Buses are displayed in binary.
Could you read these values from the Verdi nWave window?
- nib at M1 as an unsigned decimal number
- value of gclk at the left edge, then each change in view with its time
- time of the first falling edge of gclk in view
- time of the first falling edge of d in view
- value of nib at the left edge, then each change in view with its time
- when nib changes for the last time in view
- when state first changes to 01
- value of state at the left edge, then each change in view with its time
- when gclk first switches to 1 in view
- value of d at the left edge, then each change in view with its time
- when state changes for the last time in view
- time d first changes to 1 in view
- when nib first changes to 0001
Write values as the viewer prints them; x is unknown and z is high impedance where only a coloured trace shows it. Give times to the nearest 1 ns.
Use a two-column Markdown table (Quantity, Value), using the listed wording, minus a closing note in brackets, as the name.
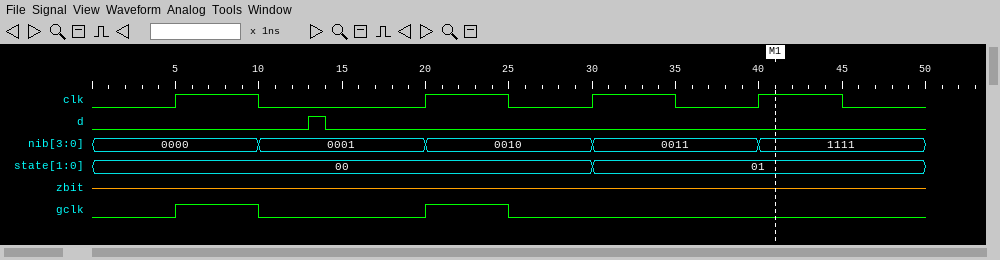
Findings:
| Quantity | Value |
|---|---|
| nib at M1 as an unsigned decimal number | 15 |
| value of gclk at the left edge, then each change in view with its time | 0, 1 at 5 ns, 0 at 10 ns, 1 at 20 ns, 0 at 25 ns |
| time of the first falling edge of gclk in view | 10 ns |
| time of the first falling edge of d in view | 14 ns |
| value of nib at the left edge, then each change in view with its time | 0000, 0001 at 10 ns, 0010 at 20 ns, 0011 at 30 ns, 1111 at 40 ns |
| when nib changes for the last time in view | 40 ns |
| when state first changes to 01 | 30 ns |
| value of state at the left edge, then each change in view with its time | 00, 01 at 30 ns |
| when gclk first switches to 1 in view | 5 ns |
| value of d at the left edge, then each change in view with its time | 0, 1 at 13 ns, 0 at 14 ns |
| when state changes for the last time in view | 30 ns |
| time d first changes to 1 in view | 13 ns |
| when nib first changes to 0001 | 10 ns |
